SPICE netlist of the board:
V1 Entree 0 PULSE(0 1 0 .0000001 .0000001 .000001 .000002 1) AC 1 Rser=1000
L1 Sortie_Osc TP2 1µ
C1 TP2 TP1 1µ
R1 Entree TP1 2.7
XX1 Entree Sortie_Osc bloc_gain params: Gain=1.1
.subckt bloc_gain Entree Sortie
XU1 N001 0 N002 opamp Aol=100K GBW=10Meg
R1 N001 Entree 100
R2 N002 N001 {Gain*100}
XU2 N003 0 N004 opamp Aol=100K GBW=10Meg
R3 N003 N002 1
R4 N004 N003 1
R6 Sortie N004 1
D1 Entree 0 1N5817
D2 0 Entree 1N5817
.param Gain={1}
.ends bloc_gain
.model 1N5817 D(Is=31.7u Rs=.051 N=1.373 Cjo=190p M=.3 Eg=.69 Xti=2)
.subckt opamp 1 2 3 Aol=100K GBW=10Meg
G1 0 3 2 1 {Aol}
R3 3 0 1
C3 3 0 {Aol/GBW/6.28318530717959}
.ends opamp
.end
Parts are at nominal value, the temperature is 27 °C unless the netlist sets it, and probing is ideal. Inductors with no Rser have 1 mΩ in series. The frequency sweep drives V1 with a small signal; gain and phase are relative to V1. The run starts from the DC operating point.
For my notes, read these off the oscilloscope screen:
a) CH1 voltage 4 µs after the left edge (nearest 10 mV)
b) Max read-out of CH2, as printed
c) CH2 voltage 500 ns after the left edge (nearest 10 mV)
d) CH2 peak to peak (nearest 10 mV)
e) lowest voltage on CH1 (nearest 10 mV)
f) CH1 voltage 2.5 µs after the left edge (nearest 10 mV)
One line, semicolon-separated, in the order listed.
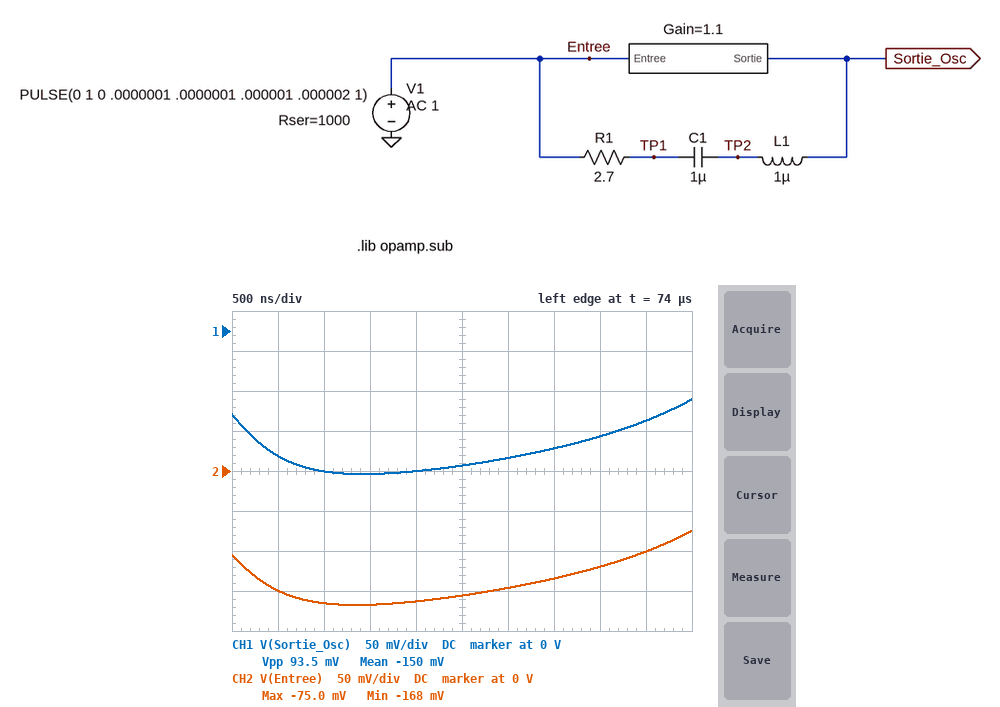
-130 mV; -75.0 mV; -150 mV; 90 mV; -180 mV; -170 mV
